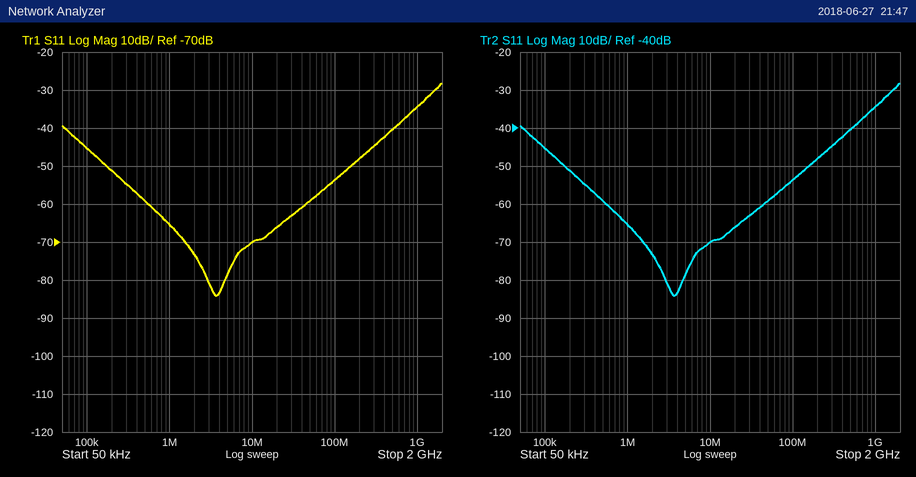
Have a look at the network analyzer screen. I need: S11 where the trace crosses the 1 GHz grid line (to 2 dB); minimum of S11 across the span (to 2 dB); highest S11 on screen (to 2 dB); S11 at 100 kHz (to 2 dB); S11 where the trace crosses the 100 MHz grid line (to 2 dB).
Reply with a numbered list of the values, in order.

1. -34 dB
2. -84 dB
3. -28 dB
4. -46 dB
5. -54 dB
